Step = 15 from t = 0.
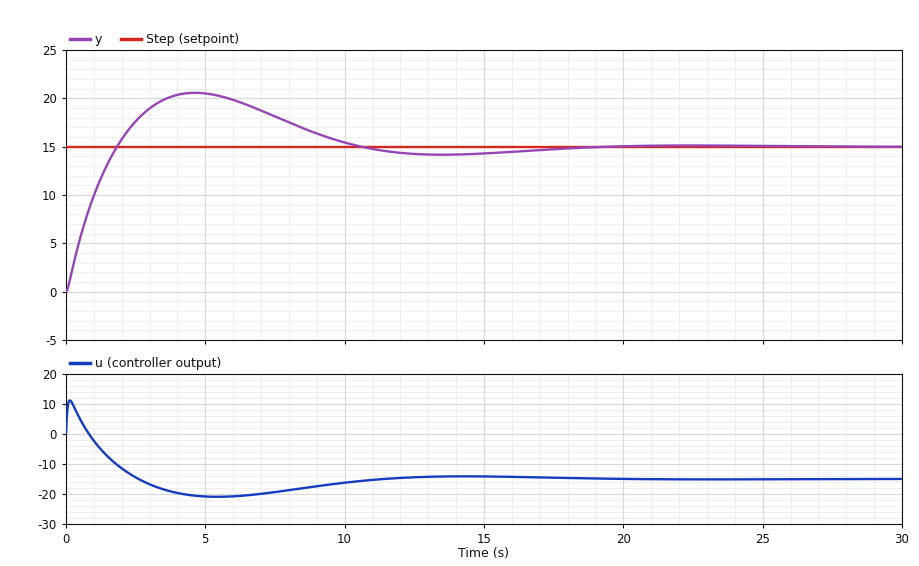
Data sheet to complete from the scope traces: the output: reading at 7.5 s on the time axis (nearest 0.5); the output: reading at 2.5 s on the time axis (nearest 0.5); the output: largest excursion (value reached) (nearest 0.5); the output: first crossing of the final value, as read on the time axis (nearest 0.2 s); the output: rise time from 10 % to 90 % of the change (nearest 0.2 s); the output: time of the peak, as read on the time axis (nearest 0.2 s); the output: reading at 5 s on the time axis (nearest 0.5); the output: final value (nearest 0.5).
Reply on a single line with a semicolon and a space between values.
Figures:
18.0; 17.5; 20.5; 1.8 s; 1.4 s; 4.6 s; 20.5; 15.0
